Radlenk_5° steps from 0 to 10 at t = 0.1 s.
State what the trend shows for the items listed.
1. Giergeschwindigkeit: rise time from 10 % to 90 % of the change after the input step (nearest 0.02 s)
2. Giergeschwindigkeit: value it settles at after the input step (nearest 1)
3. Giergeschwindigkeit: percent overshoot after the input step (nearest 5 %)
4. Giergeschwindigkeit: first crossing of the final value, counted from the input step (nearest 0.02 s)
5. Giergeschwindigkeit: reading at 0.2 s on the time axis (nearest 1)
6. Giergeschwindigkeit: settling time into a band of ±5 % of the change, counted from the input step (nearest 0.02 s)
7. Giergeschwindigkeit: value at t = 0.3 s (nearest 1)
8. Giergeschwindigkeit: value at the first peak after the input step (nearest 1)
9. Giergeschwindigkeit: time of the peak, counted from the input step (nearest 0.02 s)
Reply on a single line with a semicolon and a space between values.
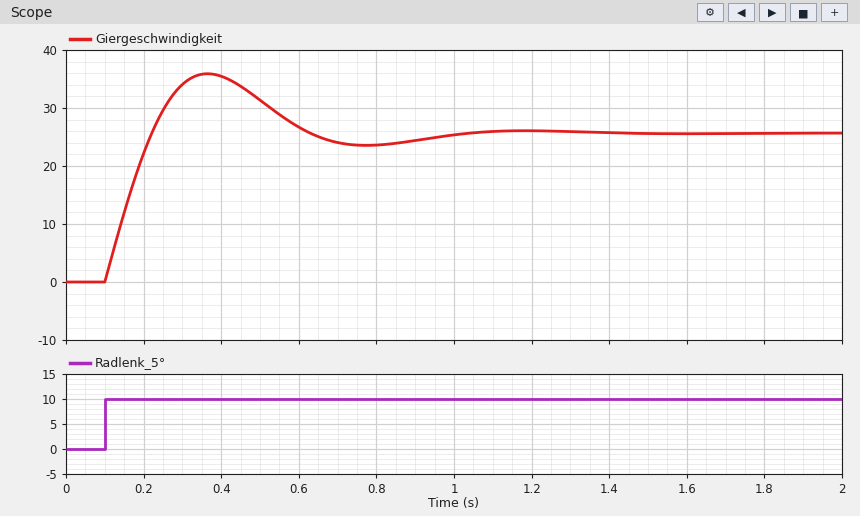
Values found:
0.10 s; 26; 40 %; 0.12 s; 22; 0.80 s; 34; 36; 0.26 s
